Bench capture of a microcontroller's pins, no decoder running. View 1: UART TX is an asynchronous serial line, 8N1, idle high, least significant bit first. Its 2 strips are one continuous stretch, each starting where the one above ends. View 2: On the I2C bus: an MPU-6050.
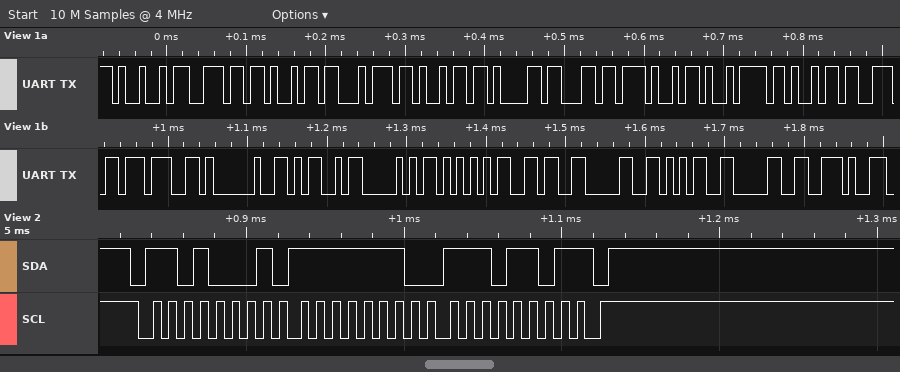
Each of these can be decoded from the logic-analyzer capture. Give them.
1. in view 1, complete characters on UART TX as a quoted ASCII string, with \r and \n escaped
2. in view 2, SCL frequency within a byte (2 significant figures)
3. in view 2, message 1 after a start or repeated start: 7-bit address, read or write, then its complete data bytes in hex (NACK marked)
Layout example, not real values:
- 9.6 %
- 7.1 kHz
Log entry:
- "Initializing MPU6050."
- 100 kHz
- 0x68 read: FE ED NACK
